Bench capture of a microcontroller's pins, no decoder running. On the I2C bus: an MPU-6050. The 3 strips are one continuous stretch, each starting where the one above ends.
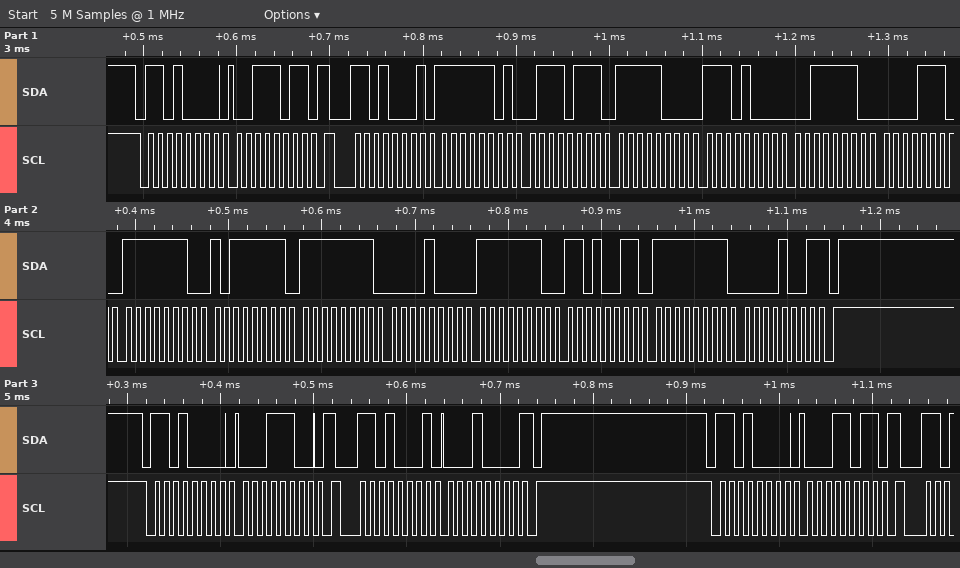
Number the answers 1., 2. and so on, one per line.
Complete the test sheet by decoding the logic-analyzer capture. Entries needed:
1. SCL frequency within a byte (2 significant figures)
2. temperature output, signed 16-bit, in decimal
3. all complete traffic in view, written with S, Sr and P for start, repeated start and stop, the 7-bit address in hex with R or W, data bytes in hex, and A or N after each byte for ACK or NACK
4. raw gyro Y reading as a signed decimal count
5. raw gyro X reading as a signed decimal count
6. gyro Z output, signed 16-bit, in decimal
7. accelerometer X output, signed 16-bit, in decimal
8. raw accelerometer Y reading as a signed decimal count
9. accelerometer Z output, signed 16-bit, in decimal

1. 100 kHz
2. -321
3. S 68W A 3B A Sr 68R A FD A 77 A F8 A E8 A 3E A 0E A FE A BF A FF A 08 A FE A D3 A FF A 09 N P S 68W A 1C A Sr 68R A 10 N P S 68W A 1B A
4. -301
5. -248
6. -247
7. -649
8. -1816
9. 15886
